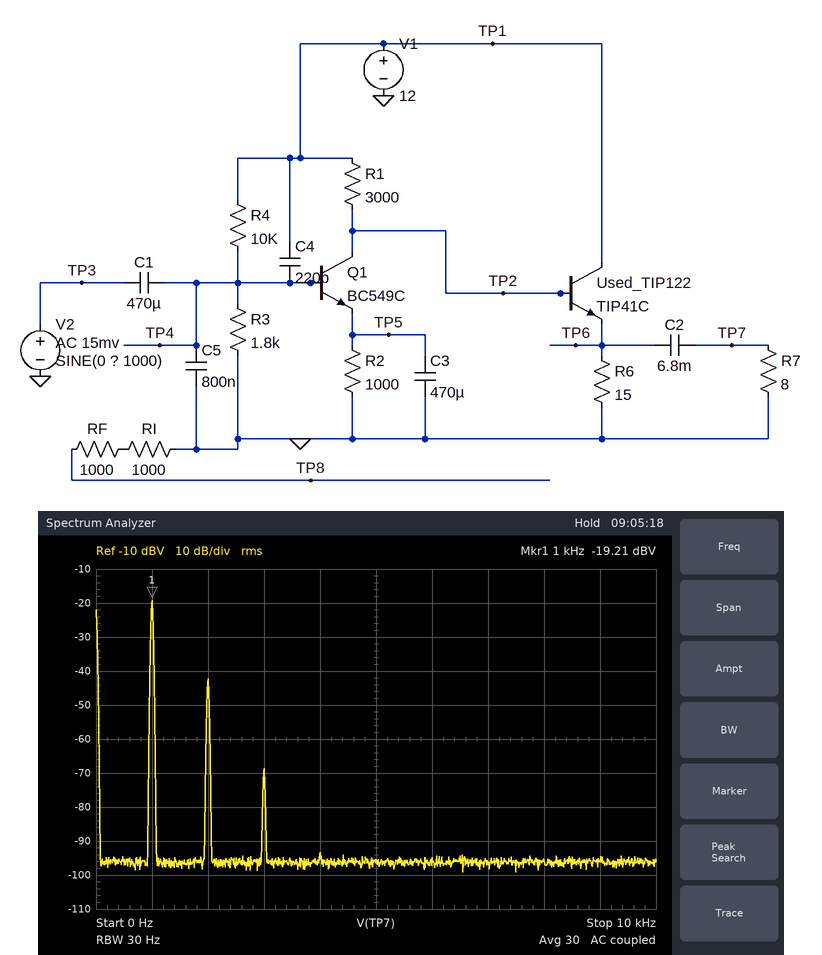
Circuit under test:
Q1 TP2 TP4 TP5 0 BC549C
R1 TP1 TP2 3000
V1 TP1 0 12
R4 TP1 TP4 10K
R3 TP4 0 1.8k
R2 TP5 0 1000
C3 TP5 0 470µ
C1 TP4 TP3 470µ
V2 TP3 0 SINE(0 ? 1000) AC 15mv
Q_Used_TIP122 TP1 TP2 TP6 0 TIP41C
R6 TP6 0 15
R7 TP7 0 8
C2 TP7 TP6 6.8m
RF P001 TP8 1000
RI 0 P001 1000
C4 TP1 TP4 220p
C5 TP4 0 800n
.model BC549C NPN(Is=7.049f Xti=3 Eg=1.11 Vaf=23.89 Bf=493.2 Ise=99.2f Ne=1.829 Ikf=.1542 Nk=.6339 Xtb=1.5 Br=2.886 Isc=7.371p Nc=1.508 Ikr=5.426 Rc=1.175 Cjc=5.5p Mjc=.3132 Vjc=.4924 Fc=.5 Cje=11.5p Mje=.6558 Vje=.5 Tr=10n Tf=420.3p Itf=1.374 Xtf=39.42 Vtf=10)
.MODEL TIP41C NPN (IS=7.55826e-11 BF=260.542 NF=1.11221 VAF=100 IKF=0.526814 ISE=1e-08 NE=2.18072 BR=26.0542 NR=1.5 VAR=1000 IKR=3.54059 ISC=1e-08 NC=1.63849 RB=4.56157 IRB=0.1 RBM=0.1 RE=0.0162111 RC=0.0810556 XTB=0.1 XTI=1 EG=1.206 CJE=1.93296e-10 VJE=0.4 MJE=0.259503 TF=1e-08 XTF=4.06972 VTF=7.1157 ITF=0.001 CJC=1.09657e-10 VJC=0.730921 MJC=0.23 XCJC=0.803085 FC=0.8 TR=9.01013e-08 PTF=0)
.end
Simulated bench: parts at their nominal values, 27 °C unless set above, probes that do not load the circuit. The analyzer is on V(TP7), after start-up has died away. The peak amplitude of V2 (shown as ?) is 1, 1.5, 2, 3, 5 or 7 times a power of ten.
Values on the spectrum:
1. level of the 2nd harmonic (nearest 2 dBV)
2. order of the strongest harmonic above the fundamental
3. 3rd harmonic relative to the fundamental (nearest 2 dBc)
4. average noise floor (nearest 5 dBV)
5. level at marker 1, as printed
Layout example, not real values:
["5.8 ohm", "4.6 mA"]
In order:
["-42 dBV", "2", "-50 dBc", "-95 dBV", "-19.21 dBV"]
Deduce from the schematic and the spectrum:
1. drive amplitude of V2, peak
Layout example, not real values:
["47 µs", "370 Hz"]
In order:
["7 mV"]
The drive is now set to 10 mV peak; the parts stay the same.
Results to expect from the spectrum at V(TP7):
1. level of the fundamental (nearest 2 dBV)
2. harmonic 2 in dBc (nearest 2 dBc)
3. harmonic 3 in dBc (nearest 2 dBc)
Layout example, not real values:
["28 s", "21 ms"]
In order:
["-16 dBV", "-20 dBc", "-44 dBc"]
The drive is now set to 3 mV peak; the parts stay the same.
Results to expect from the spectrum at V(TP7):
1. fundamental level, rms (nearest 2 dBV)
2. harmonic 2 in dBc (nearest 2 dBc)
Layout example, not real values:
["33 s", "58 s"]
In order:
["-26 dBV", "-30 dBc"]
